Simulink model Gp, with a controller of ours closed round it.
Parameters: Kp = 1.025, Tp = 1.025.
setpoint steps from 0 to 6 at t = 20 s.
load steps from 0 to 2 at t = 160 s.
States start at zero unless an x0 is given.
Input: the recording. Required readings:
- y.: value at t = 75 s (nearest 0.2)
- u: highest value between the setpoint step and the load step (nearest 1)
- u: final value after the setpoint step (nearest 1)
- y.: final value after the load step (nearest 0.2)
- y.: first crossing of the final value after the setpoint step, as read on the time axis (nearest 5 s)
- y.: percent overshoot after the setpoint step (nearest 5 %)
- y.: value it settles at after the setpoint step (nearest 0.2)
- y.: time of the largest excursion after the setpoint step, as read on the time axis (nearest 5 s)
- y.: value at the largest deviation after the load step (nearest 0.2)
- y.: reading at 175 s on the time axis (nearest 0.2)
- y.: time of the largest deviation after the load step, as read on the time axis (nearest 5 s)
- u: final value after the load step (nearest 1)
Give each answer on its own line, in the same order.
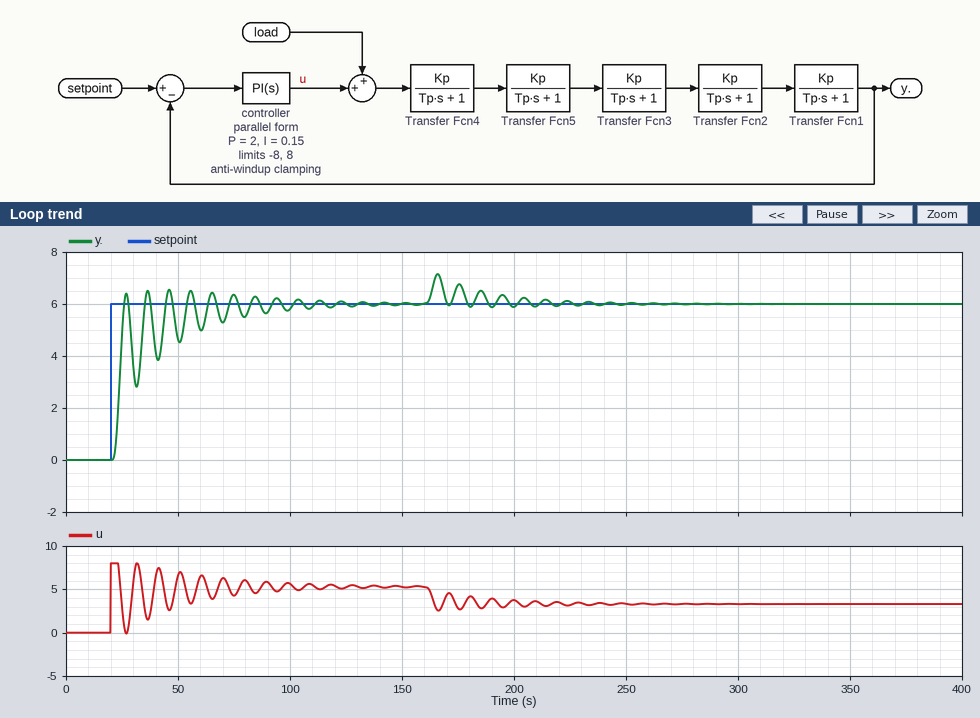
6.4
8
5
6.0
25 s
10 %
6.0
45 s
7.2
6.8
165 s
3
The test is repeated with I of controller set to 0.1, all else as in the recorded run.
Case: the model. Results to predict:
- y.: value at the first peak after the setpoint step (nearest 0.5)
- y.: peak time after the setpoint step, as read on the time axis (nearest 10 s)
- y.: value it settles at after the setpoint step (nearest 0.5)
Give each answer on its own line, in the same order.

6.5
30 s
6.0
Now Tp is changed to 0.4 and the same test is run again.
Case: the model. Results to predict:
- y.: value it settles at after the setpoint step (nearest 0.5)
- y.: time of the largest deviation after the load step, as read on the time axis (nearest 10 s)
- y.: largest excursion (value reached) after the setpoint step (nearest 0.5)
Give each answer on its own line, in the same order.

6.0
160 s
6.5
